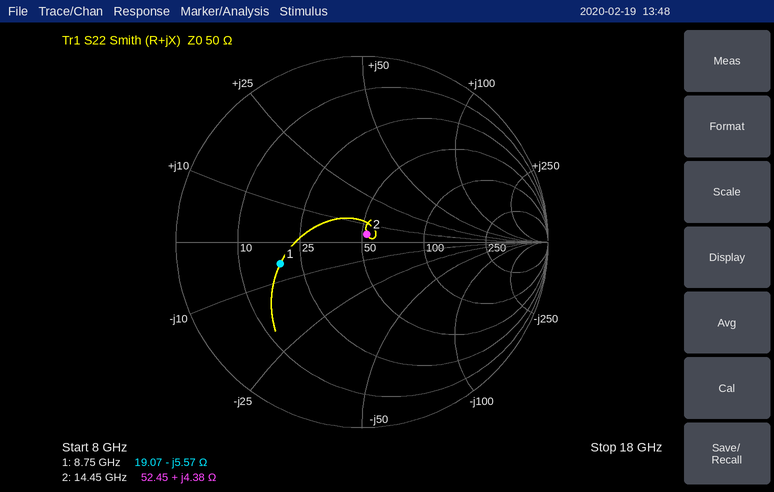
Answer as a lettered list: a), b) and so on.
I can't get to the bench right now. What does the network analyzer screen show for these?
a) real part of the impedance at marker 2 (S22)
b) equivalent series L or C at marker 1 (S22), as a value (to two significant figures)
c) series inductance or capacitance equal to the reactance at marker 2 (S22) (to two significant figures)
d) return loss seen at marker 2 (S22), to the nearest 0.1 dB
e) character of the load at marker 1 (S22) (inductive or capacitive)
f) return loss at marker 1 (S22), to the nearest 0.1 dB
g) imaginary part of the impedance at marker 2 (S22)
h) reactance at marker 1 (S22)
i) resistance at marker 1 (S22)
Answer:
a) 52.45 Ω
b) 3.3 pF
c) 48 pH
d) 26.2 dB
e) capacitive
f) 6.9 dB
g) +4.38 Ω
h) -5.57 Ω
i) 19.07 Ω
